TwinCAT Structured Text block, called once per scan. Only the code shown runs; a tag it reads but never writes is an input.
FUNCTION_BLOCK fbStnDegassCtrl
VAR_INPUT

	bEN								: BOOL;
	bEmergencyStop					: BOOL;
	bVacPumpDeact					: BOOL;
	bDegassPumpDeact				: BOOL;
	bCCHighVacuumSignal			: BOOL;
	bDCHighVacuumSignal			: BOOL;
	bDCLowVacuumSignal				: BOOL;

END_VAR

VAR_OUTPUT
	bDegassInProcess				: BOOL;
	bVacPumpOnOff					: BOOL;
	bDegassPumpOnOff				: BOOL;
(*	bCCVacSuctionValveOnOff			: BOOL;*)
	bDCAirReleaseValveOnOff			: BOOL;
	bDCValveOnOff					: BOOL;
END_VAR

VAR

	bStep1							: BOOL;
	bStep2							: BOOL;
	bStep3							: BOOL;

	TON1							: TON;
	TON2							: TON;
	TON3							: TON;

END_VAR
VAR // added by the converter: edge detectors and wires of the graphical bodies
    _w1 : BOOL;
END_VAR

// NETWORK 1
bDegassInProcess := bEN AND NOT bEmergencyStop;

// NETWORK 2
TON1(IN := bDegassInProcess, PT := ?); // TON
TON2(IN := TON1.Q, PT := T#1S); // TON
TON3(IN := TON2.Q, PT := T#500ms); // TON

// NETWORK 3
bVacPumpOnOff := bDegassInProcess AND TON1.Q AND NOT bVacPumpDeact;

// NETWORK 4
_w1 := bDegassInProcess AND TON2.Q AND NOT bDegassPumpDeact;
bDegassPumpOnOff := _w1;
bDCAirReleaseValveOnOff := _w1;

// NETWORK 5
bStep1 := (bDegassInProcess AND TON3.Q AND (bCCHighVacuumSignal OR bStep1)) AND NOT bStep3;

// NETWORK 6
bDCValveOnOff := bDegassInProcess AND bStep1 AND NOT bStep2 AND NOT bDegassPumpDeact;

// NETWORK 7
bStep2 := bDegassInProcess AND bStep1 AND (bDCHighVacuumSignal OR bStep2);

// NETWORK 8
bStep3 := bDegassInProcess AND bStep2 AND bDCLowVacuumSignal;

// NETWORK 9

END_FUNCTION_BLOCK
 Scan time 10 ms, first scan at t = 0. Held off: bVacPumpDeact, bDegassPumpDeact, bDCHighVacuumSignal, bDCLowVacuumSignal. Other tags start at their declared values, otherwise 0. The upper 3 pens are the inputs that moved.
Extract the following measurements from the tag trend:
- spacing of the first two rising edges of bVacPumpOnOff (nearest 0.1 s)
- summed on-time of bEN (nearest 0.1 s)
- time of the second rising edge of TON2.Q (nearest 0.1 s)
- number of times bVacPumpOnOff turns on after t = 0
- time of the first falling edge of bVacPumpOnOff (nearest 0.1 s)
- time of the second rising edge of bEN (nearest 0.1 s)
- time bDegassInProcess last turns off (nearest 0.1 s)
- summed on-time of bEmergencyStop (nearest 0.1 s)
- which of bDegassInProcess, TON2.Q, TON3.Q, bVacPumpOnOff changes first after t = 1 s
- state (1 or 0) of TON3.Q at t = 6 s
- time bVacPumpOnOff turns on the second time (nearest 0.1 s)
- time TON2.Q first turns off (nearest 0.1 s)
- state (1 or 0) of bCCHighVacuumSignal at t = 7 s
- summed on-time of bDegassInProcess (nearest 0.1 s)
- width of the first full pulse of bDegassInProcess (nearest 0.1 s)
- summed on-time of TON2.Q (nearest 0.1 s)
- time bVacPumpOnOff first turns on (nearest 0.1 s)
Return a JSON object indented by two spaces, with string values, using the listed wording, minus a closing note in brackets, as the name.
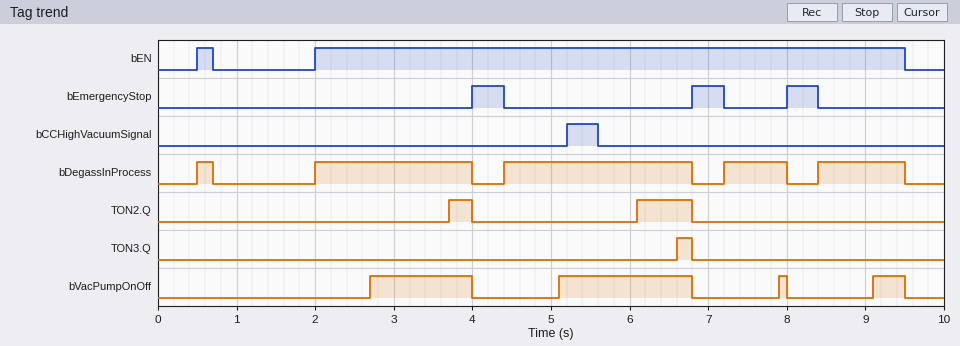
{
  "spacing of the first two rising edges of bVacPumpOnOff": "2.4 s",
  "summed on-time of bEN": "7.7 s",
  "time of the second rising edge of TON2.Q": "6.1 s",
  "number of times bVacPumpOnOff turns on after t = 0": "4",
  "time of the first falling edge of bVacPumpOnOff": "4.0 s",
  "time of the second rising edge of bEN": "2.0 s",
  "time bDegassInProcess last turns off": "9.5 s",
  "summed on-time of bEmergencyStop": "1.2 s",
  "which of bDegassInProcess, TON2.Q, TON3.Q, bVacPumpOnOff changes first after t = 1 s": "bDegassInProcess",
  "state (1 or 0) of TON3.Q at t = 6 s": "0",
  "time bVacPumpOnOff turns on the second time": "5.1 s",
  "time TON2.Q first turns off": "4.0 s",
  "state (1 or 0) of bCCHighVacuumSignal at t = 7 s": "0",
  "summed on-time of bDegassInProcess": "6.5 s",
  "width of the first full pulse of bDegassInProcess": "0.2 s",
  "summed on-time of TON2.Q": "1.0 s",
  "time bVacPumpOnOff first turns on": "2.7 s"
}
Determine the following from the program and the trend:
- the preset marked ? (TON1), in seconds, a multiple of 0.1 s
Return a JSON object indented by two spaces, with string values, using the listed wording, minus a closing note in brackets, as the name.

{
  "the preset marked ? (TON1), in seconds, a multiple of 0.1 s": "0.7 s"
}
